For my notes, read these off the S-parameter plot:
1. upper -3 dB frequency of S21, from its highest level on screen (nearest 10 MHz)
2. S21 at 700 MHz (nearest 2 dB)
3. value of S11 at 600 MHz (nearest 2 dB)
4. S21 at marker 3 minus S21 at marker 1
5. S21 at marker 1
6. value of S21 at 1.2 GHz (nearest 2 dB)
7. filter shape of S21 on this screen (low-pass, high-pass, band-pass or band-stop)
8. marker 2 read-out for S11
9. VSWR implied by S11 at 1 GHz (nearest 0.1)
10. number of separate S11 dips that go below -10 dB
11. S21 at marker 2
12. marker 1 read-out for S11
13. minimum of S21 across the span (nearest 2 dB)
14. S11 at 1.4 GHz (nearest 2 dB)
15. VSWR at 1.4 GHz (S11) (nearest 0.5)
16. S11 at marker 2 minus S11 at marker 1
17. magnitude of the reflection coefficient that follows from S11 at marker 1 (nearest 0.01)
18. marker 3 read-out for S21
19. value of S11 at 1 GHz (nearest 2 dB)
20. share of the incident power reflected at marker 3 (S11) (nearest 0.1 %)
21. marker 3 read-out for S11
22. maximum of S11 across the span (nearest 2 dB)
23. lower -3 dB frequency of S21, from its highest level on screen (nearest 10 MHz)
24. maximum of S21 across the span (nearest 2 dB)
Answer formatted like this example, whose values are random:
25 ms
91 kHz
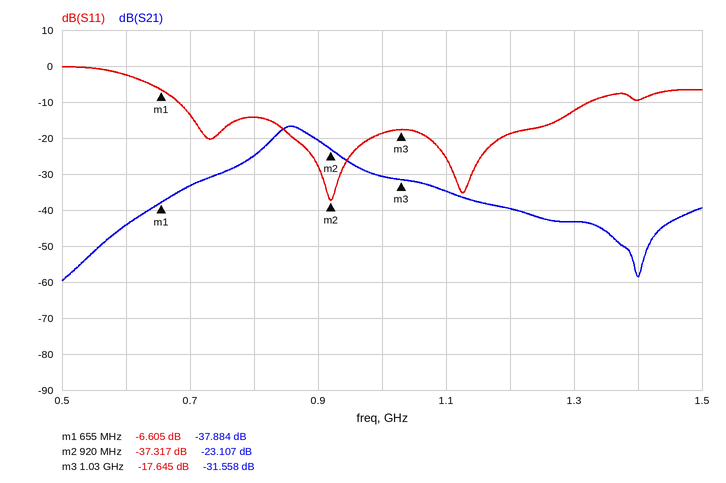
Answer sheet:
890 MHz
-34 dB
-2 dB
6.326 dB
-37.884 dB
-40 dB
band-pass
-37.317 dB
1.3
3
-23.107 dB
-6.605 dB
-60 dB
-10 dB
2.0
-30.712 dB
0.47
-31.558 dB
-18 dB
1.7 %
-17.645 dB
0 dB
830 MHz
-16 dB
